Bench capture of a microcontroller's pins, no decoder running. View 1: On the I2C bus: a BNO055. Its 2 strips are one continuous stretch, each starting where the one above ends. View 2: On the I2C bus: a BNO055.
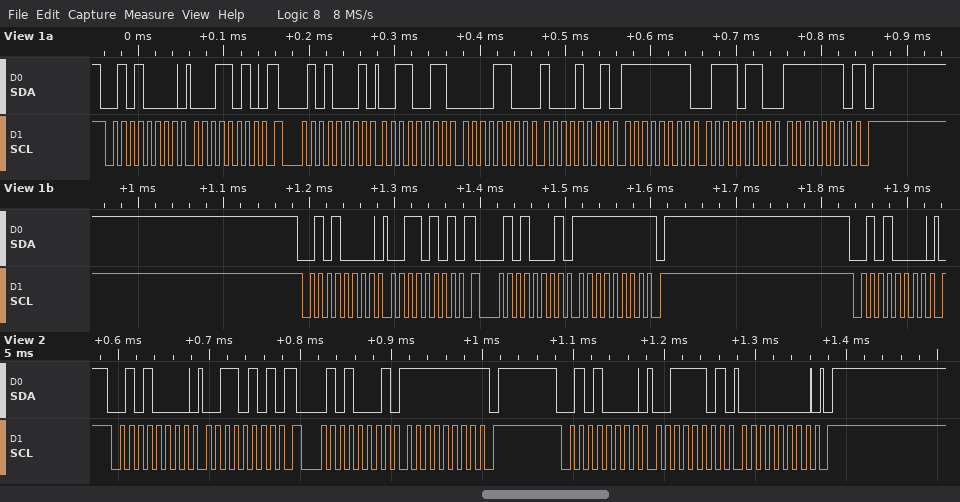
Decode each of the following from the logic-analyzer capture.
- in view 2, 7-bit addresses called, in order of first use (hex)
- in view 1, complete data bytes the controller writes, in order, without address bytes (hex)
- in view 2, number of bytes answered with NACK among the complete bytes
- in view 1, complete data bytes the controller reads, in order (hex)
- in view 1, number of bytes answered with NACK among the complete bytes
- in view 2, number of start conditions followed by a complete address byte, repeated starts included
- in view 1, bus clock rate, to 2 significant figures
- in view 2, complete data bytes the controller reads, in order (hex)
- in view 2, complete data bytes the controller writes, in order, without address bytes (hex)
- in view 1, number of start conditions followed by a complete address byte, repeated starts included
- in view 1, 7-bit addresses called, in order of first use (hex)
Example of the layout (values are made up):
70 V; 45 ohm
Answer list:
0x28; 1A 35; 1; 33 0C 89 FF 76 FE FF; 2; 3; 100 kHz; FF; 35 3D 00; 5; 0x28
